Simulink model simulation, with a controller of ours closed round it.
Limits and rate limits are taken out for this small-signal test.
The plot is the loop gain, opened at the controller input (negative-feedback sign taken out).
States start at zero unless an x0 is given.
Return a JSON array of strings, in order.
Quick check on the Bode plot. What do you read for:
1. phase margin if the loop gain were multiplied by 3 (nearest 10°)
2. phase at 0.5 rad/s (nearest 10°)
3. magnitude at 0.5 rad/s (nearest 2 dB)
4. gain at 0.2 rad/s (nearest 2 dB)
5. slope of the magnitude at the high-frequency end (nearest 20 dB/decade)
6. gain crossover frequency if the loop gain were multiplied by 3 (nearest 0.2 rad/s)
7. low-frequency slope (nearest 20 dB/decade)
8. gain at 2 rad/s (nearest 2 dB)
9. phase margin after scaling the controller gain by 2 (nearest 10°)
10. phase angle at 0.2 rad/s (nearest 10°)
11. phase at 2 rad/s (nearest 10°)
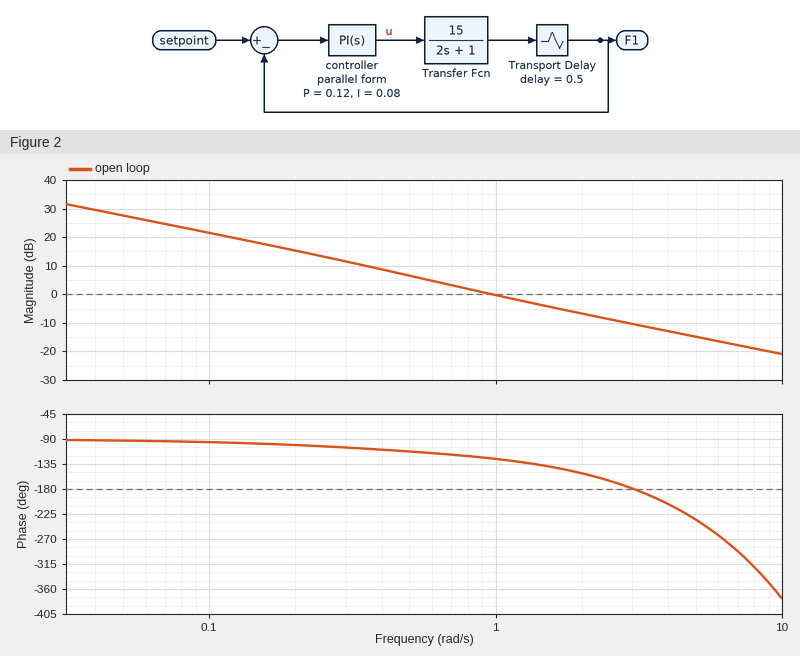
["10°", "-110°", "6 dB", "16 dB", "-20 dB/decade", "2.8 rad/s", "-20 dB/decade", "-6 dB", "30°", "-100°", "-150°"]
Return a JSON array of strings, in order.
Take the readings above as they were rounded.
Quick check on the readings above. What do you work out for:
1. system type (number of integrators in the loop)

["1"]
